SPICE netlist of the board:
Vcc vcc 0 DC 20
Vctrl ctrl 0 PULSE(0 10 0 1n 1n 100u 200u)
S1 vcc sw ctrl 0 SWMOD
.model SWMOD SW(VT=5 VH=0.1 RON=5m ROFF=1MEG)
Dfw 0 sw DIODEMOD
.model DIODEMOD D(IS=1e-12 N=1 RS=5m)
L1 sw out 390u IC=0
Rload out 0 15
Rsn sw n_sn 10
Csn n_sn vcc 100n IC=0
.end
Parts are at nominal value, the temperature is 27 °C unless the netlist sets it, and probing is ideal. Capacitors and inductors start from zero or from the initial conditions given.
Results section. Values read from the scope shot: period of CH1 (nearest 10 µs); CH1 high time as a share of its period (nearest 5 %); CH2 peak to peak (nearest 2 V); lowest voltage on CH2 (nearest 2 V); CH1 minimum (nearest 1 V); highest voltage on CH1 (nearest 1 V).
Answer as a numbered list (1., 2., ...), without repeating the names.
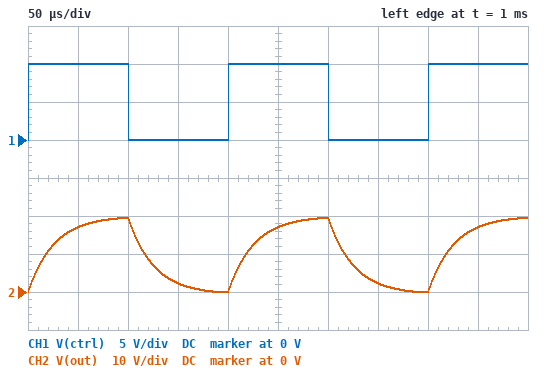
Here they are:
1. 200 µs
2. 50 %
3. 20 V
4. 0 V
5. 0 V
6. 10 V
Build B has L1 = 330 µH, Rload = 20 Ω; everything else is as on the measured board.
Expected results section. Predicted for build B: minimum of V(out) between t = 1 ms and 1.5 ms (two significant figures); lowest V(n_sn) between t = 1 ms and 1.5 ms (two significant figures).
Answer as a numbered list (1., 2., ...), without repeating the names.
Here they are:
1. -130 mV
2. -700 mV
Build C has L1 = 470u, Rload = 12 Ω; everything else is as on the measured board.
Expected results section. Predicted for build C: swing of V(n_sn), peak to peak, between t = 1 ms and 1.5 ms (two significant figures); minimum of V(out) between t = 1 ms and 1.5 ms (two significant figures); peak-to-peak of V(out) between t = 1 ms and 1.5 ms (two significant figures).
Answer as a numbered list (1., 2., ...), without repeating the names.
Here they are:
1. 21 V
2. 820 mV
3. 18 V
